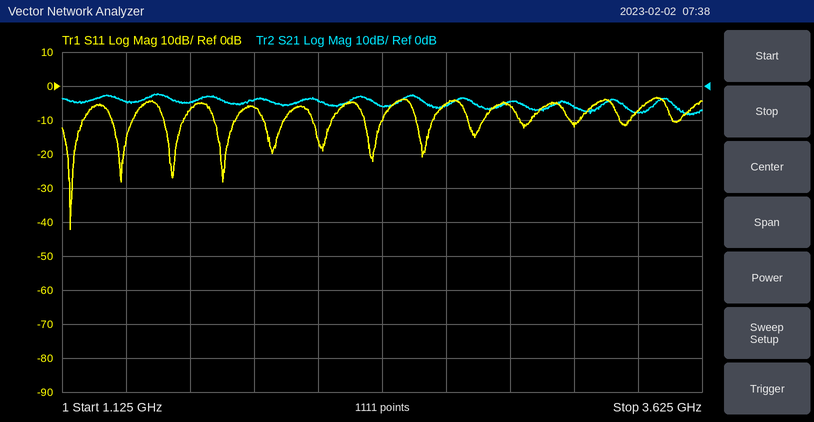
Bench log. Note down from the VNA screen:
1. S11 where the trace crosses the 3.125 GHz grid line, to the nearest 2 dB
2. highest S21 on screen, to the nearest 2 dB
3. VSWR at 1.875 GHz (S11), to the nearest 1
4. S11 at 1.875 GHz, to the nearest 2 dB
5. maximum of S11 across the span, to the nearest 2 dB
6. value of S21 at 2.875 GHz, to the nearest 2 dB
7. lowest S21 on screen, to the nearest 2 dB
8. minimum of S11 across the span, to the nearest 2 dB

-12 dB
-2 dB
3
-6 dB
-4 dB
-4 dB
-8 dB
-42 dB
